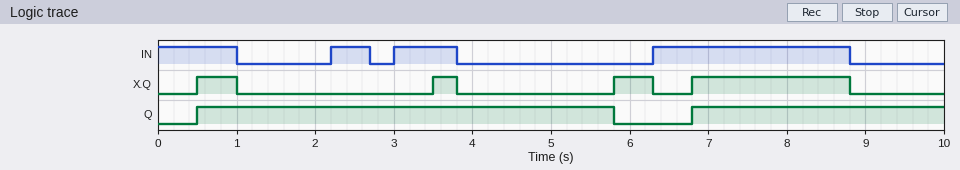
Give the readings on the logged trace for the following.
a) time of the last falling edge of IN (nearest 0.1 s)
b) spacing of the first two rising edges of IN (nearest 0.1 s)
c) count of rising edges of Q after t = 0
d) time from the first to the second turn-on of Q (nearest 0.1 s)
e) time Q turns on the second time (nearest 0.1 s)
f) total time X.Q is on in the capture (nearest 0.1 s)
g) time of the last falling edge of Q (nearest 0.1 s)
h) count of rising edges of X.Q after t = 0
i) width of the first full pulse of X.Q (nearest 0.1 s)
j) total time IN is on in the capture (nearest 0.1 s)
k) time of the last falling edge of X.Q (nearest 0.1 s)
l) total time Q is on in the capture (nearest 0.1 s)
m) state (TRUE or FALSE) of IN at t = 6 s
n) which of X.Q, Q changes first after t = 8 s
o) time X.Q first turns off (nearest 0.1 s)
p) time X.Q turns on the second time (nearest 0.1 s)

8.8 s
0.8 s
2
6.3 s
6.8 s
3.3 s
5.8 s
4
0.5 s
4.8 s
8.8 s
8.5 s
FALSE
X.Q
1.0 s
3.5 s
